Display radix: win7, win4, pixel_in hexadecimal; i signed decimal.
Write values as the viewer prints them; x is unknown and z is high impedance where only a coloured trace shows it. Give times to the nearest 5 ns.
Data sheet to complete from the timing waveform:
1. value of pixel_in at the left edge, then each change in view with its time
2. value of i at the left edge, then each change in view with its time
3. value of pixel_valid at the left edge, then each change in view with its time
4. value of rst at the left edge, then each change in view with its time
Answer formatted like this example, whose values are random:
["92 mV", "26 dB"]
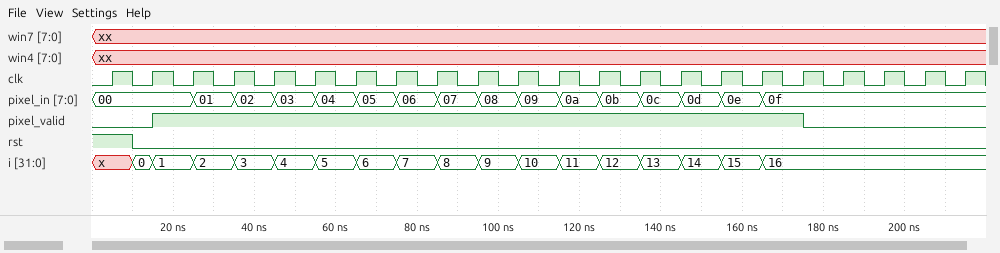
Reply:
["00, 01 at 25 ns, 02 at 35 ns, 03 at 45 ns, 04 at 55 ns, 05 at 65 ns, 06 at 75 ns, 07 at 85 ns, 08 at 95 ns, 09 at 105 ns, 0a at 115 ns, 0b at 125 ns, 0c at 135 ns, 0d at 145 ns, 0e at 155 ns, 0f at 165 ns", "x, 0 at 10 ns, 1 at 15 ns, 2 at 25 ns, 3 at 35 ns, 4 at 45 ns, 5 at 55 ns, 6 at 65 ns, 7 at 75 ns, 8 at 85 ns, 9 at 95 ns, 10 at 105 ns, 11 at 115 ns, 12 at 125 ns, 13 at 135 ns, 14 at 145 ns, 15 at 155 ns, 16 at 165 ns", "0, 1 at 15 ns, 0 at 175 ns", "1, 0 at 10 ns"]
